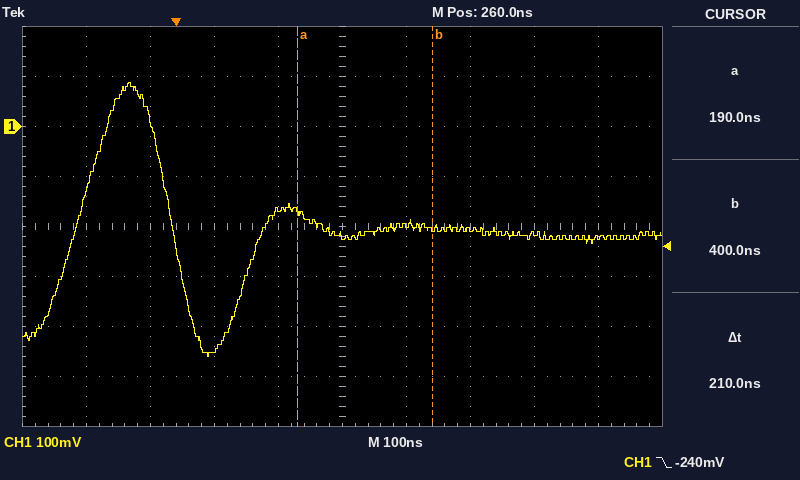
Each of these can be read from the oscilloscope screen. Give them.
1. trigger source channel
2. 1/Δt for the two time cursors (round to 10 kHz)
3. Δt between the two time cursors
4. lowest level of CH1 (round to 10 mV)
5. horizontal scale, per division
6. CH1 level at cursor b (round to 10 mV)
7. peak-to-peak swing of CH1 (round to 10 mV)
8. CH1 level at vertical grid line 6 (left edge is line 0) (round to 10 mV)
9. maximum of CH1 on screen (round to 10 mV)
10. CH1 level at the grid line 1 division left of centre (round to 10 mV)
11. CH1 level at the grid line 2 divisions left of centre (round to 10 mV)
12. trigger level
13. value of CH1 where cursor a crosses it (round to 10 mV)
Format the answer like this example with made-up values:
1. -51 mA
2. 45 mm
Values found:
1. CH1
2. 4.76 MHz
3. 210 ns
4. -460 mV
5. 100 ns
6. -200 mV
7. 550 mV
8. -200 mV
9. 90 mV
10. -170 mV
11. -450 mV
12. -240 mV
13. -170 mV
